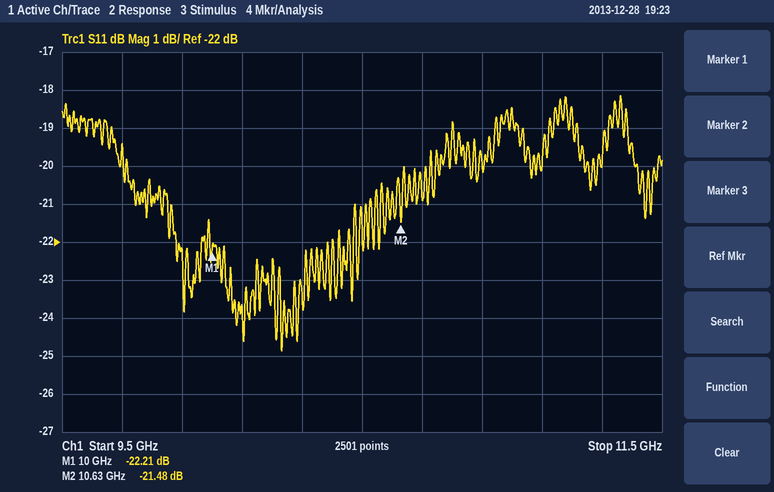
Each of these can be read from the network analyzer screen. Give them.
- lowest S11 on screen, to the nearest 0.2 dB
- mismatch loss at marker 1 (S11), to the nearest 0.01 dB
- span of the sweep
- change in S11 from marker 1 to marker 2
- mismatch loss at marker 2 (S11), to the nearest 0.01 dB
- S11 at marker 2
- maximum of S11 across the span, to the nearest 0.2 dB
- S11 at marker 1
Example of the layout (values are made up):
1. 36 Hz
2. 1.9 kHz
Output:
1. -24.8 dB
2. 0.03 dB
3. 2 GHz
4. 0.73 dB
5. 0.03 dB
6. -21.48 dB
7. -18.2 dB
8. -22.21 dB
